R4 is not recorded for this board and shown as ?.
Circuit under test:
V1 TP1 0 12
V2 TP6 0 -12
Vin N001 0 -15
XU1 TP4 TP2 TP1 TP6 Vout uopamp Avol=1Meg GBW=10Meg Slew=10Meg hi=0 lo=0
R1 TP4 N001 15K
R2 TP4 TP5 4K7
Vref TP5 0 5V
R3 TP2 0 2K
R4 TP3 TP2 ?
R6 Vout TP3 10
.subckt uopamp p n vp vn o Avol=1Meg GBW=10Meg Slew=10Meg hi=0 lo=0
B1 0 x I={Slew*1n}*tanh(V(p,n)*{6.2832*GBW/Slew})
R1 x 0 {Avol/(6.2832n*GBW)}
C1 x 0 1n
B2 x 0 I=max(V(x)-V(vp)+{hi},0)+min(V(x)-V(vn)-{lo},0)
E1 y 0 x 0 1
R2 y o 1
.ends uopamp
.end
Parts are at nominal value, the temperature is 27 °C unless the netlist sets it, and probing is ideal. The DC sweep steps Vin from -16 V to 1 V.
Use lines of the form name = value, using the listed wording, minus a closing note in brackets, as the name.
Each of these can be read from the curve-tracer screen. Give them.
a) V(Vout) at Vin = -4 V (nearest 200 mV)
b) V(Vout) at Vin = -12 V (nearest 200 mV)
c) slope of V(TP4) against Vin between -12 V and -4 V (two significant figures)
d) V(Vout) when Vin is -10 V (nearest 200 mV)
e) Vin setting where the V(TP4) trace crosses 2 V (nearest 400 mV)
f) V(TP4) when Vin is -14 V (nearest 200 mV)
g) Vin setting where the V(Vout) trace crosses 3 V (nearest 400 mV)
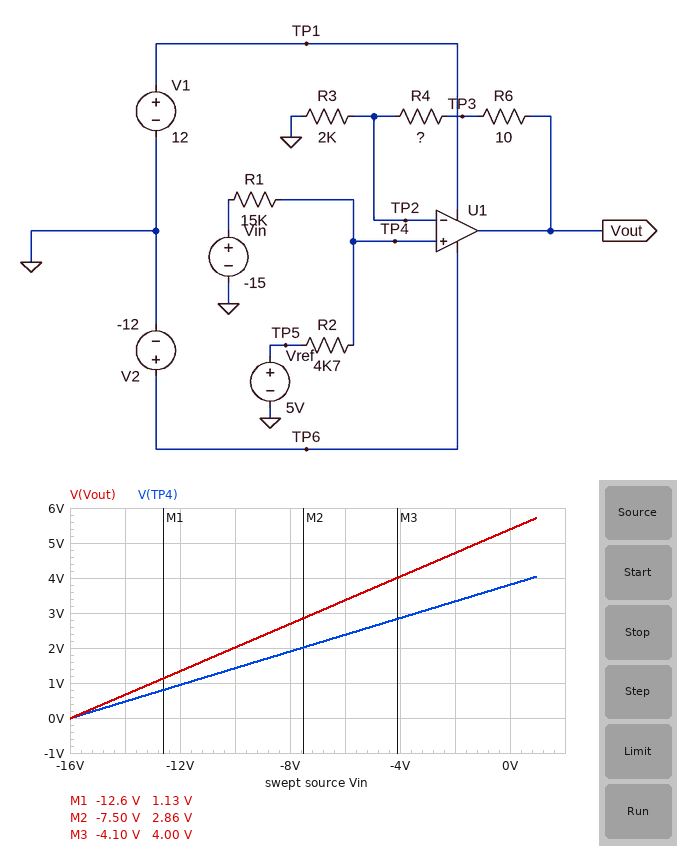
V(Vout) at Vin = -4 V = 4.0 V
V(Vout) at Vin = -12 V = 1.4 V
slope of V(TP4) against Vin between -12 V and -4 V = 0.24 V/V
V(Vout) when Vin is -10 V = 2.0 V
Vin setting where the V(TP4) trace crosses 2 V = -7.6 V
V(TP4) when Vin is -14 V = 400 mV
Vin setting where the V(Vout) trace crosses 3 V = -7.2 V
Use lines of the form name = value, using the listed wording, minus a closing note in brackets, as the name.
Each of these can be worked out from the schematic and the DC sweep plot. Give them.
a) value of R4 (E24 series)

value of R4 = 820 Ω
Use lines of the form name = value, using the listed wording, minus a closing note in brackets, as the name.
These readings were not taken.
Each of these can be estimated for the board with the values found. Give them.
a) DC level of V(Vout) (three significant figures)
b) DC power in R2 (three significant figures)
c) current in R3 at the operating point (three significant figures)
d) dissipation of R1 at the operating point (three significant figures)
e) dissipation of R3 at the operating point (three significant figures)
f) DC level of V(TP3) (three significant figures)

DC level of V(Vout) = 323 mV
DC power in R2 = 4.84 mW
current in R3 at the operating point = 114 µA
dissipation of R1 at the operating point = 15.5 mW
dissipation of R3 at the operating point = 26.1 µW
DC level of V(TP3) = 322 mV
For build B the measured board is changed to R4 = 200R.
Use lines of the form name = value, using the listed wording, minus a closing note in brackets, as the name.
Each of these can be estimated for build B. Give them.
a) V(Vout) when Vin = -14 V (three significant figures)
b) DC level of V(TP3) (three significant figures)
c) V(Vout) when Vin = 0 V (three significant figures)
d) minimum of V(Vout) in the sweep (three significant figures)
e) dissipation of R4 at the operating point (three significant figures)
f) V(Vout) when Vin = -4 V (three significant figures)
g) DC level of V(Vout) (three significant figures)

V(Vout) when Vin = -14 V = 516 mV
DC level of V(TP3) = 251 mV
V(Vout) when Vin = 0 V = 4.21 V
minimum of V(Vout) in the sweep = -11.2 mV
dissipation of R4 at the operating point = 2.61 µW
V(Vout) when Vin = -4 V = 3.15 V
DC level of V(Vout) = 252 mV
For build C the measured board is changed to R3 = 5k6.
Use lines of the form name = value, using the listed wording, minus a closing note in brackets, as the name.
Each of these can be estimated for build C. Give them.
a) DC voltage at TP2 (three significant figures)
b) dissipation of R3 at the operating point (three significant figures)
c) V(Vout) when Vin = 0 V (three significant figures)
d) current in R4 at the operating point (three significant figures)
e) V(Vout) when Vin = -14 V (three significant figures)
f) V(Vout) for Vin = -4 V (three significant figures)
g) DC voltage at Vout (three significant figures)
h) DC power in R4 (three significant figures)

DC voltage at TP2 = 228 mV
dissipation of R3 at the operating point = 9.32 µW
V(Vout) when Vin = 0 V = 4.37 V
current in R4 at the operating point = 40.8 µA
V(Vout) when Vin = -14 V = 536 mV
V(Vout) for Vin = -4 V = 3.28 V
DC voltage at Vout = 262 mV
DC power in R4 = 1.36 µW
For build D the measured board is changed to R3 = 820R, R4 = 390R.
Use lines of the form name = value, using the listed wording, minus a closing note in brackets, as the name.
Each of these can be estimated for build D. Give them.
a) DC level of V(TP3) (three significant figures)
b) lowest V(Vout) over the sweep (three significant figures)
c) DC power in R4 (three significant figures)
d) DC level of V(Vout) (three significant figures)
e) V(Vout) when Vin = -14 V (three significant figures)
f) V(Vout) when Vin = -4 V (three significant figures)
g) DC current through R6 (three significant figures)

DC level of V(TP3) = 337 mV
lowest V(Vout) over the sweep = -15.1 mV
DC power in R4 = 30.3 µW
DC level of V(Vout) = 340 mV
V(Vout) when Vin = -14 V = 695 mV
V(Vout) when Vin = -4 V = 4.24 V
DC current through R6 = 279 µA
